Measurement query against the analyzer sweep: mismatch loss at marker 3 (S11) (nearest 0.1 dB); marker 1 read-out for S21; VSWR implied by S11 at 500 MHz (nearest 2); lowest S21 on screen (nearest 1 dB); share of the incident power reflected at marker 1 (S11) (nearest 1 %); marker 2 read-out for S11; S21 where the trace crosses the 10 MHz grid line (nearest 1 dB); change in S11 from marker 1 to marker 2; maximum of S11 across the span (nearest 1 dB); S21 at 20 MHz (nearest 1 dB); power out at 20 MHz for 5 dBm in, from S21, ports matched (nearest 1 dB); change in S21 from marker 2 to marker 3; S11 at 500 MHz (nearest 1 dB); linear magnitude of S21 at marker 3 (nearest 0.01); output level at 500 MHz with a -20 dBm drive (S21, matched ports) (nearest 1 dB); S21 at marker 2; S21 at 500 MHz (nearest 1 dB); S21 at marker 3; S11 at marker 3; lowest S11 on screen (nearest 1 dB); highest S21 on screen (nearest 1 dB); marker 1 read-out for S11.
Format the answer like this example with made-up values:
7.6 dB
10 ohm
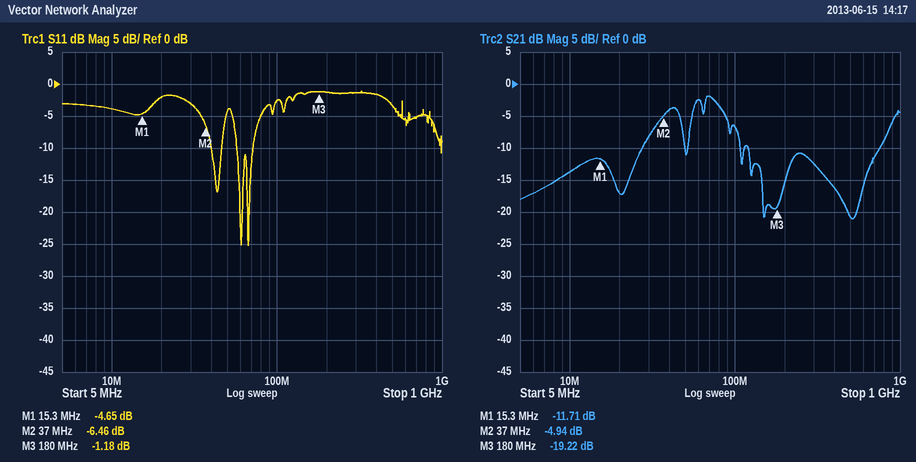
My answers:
6.2 dB
-11.71 dB
6
-21 dB
34 %
-6.46 dB
-14 dB
-1.81 dB
-1 dB
-17 dB
-12 dBm
-14.28 dB
-3 dB
0.11
-41 dBm
-4.94 dB
-21 dB
-19.22 dB
-1.18 dB
-25 dB
-2 dB
-4.65 dB
